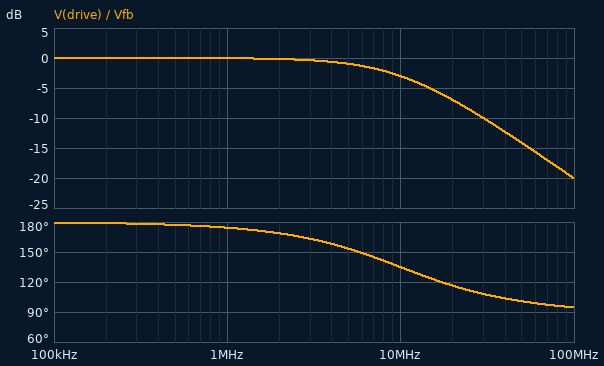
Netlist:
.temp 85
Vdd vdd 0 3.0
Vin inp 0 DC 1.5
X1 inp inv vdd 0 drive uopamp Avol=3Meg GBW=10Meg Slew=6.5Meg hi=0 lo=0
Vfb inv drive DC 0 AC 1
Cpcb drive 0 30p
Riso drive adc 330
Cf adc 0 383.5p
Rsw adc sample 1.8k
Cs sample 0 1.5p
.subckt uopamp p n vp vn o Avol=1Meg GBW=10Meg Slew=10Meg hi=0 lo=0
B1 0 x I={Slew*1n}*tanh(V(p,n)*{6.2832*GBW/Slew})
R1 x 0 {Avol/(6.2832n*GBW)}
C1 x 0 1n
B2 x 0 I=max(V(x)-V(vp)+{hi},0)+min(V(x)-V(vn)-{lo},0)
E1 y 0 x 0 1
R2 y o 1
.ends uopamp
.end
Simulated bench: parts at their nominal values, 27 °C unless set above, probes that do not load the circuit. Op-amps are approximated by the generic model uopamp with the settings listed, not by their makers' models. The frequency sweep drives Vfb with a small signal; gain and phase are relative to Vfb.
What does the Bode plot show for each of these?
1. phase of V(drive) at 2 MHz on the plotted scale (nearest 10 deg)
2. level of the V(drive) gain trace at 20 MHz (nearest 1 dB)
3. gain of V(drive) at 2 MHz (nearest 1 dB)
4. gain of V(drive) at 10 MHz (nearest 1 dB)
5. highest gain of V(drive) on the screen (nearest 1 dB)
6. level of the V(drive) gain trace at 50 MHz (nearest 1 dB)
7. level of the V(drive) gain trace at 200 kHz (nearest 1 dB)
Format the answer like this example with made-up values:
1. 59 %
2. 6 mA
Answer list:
1. 170 deg
2. -7 dB
3. 0 dB
4. -3 dB
5. 0 dB
6. -14 dB
7. 0 dB
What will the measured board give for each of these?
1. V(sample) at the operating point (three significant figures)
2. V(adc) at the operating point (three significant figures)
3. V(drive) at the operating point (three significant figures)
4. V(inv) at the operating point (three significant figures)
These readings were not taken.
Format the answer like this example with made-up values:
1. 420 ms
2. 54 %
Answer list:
1. 1.50 V
2. 1.50 V
3. 1.50 V
4. 1.50 V
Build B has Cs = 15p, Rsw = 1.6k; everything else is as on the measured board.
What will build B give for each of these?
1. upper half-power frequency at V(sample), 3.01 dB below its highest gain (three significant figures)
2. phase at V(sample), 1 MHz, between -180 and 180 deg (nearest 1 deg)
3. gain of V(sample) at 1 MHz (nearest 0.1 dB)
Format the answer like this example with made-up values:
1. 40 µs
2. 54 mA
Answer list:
1. 1.15 MHz
2. 126 deg
3. -2.4 dB
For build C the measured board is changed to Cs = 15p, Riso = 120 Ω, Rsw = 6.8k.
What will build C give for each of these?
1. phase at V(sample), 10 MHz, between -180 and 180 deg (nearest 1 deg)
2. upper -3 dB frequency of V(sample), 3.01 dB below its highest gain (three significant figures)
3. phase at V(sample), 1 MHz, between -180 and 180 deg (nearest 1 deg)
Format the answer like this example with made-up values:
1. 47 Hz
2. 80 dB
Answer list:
1. -17 deg
2. 1.30 MHz
3. 125 deg
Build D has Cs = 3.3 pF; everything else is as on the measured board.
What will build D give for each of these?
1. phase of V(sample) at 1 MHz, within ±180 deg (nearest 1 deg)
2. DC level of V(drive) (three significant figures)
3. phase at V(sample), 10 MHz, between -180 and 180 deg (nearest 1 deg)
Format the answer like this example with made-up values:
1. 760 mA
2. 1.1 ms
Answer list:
1. 133 deg
2. 1.50 V
3. 32 deg
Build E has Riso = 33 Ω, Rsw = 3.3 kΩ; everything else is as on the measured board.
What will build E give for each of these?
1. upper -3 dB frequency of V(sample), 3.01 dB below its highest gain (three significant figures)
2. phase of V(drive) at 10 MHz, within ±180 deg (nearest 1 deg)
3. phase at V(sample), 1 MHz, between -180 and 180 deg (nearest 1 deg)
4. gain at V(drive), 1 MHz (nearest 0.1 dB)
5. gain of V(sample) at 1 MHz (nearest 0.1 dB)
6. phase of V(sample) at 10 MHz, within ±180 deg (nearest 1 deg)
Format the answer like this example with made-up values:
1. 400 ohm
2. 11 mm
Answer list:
1. 6.91 MHz
2. 134 deg
3. 168 deg
4. 0 dB
5. -0.1 dB
6. 78 deg
